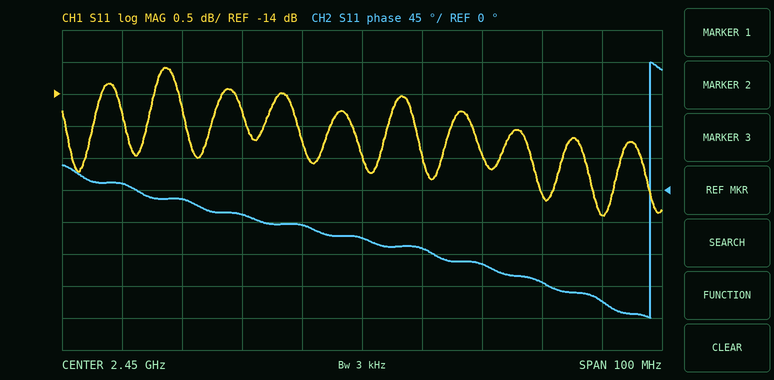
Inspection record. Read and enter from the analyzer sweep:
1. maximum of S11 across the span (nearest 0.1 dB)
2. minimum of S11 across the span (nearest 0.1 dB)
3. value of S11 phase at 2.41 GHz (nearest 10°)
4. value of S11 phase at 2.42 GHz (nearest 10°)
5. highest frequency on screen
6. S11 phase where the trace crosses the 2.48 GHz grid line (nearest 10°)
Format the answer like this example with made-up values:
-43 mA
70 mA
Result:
-13.6 dB
-15.9 dB
10°
-10°
2.5 GHz
-130°
